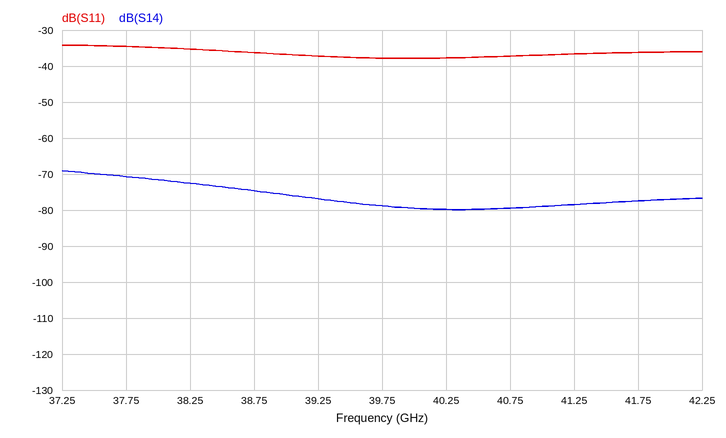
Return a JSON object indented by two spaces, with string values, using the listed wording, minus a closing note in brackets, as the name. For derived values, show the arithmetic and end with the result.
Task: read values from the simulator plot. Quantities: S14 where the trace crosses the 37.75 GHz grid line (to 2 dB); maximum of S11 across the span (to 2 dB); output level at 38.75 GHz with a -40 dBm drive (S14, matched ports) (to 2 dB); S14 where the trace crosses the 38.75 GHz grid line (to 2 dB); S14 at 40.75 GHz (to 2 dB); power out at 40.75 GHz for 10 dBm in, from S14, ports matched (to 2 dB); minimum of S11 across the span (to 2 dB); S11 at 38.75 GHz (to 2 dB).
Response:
{
  "S14 where the trace crosses the 37.75 GHz grid line": "-70 dB",
  "maximum of S11 across the span": "-34 dB",
  "output level at 38.75 GHz with a -40 dBm drive (S14, matched ports)": "-40 dBm + (-74 dB) = -114 dBm",
  "S14 where the trace crosses the 38.75 GHz grid line": "-74 dB",
  "S14 at 40.75 GHz": "-80 dB",
  "power out at 40.75 GHz for 10 dBm in, from S14, ports matched": "10 dBm + (-80 dB) = -70 dBm",
  "minimum of S11 across the span": "-38 dB",
  "S11 at 38.75 GHz": "-36 dB"
}
